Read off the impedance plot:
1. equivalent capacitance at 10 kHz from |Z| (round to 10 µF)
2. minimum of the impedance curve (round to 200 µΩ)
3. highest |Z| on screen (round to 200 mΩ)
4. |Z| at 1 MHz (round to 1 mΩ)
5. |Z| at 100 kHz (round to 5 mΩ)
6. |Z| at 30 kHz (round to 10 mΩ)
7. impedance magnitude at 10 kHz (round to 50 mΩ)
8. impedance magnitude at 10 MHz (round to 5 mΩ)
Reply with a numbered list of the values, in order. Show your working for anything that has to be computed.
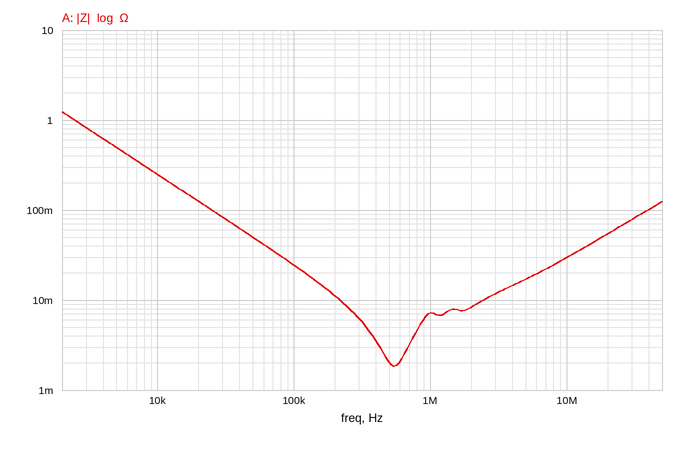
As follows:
1. C = 1/(2π × 10 kHz × 250 mΩ) ≈ 63.7 µF, so 60 µF to the nearest 10 µF
2. 1.8 mΩ
3. 1.2 Ω
4. 7 mΩ
5. 25 mΩ
6. 80 mΩ
7. 250 mΩ
8. 30 mΩ
